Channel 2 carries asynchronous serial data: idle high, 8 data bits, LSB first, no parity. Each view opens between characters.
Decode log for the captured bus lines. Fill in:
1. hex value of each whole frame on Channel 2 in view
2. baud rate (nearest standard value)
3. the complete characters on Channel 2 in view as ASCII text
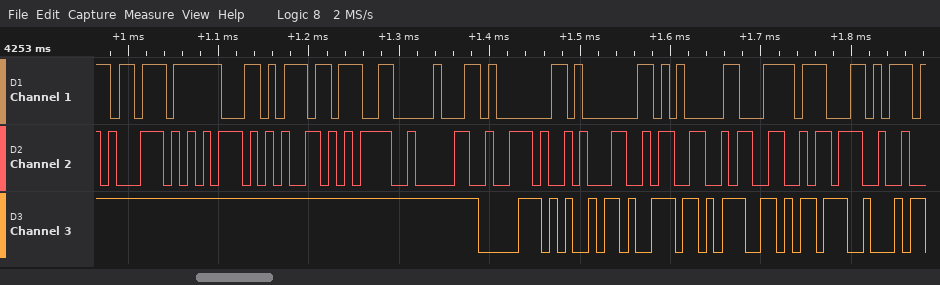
71, 75, 65, 3D, 30, 2E, 31, 33, 33, 3B
115200 baud
"que=0.133;"
